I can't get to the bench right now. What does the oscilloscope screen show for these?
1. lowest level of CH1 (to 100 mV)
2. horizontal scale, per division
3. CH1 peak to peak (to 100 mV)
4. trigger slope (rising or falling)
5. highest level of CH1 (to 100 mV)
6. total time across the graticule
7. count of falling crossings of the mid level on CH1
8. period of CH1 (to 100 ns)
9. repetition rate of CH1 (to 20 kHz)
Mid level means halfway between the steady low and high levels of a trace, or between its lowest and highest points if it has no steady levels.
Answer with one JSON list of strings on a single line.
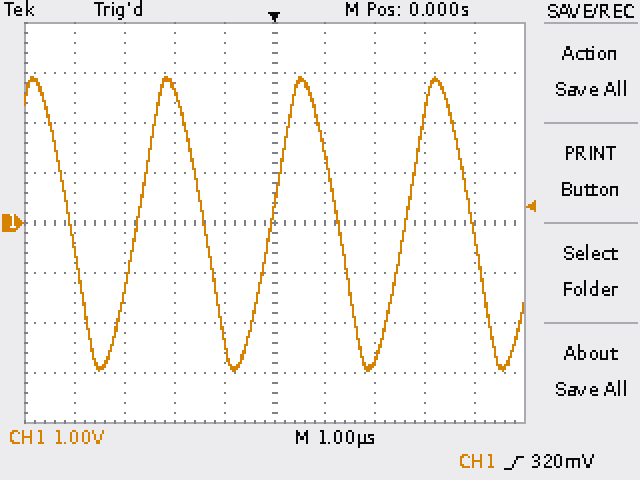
["-3.0 V", "1 µs", "5.9 V", "rising", "2.9 V", "10 µs", "4", "2.7 µs", "380 kHz"]
